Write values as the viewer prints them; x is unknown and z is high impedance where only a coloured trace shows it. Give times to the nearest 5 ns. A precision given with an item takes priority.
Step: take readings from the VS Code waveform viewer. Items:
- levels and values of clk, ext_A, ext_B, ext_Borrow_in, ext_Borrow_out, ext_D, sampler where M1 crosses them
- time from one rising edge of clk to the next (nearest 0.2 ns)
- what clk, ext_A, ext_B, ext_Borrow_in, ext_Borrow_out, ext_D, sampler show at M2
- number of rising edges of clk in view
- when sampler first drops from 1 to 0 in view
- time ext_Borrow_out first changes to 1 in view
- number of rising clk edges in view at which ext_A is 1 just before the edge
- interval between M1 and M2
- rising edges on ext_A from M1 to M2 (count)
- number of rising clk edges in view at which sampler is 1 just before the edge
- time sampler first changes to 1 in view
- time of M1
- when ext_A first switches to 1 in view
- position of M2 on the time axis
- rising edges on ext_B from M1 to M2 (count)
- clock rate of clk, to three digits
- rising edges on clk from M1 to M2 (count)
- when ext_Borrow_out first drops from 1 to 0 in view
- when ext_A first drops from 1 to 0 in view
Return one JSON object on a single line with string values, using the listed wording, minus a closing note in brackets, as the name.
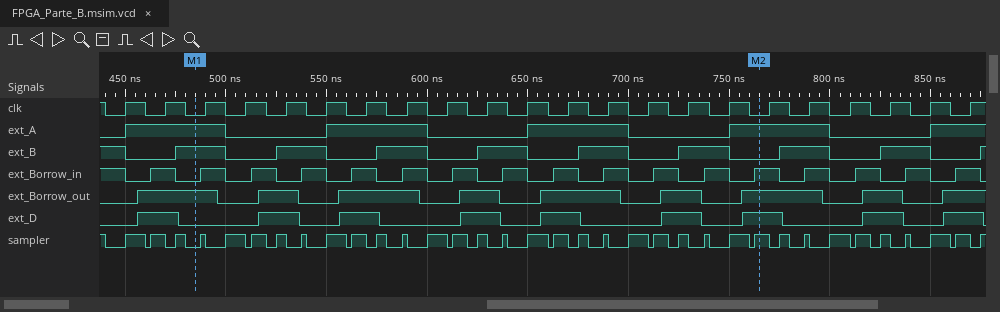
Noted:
{"levels and values of clk, ext_A, ext_B, ext_Borrow_in, ext_Borrow_out, ext_D, sampler where M1 crosses them": "clk=0, ext_A=1, ext_B=1, ext_Borrow_in=0, ext_Borrow_out=1, ext_D=0, sampler=0", "time from one rising edge of clk to the next": "20 ns", "what clk, ext_A, ext_B, ext_Borrow_in, ext_Borrow_out, ext_D, sampler show at M2": "clk=0, ext_A=1, ext_B=0, ext_Borrow_in=1, ext_Borrow_out=1, ext_D=1, sampler=1", "number of rising edges of clk in view": "22", "when sampler first drops from 1 to 0 in view": "440 ns", "time ext_Borrow_out first changes to 1 in view": "455 ns", "number of rising clk edges in view at which ext_A is 1 just before the edge": "9", "interval between M1 and M2": "280 ns", "rising edges on ext_A from M1 to M2": "3", "number of rising clk edges in view at which sampler is 1 just before the edge": "17", "time sampler first changes to 1 in view": "450 ns", "time of M1": "485 ns", "when ext_A first switches to 1 in view": "450 ns", "position of M2 on the time axis": "765 ns", "rising edges on ext_B from M1 to M2": "5", "clock rate of clk, to three digits": "50.0 MHz", "rising edges on clk from M1 to M2": "14", "when ext_Borrow_out first drops from 1 to 0 in view": "495 ns", "when ext_A first drops from 1 to 0 in view": "500 ns"}
